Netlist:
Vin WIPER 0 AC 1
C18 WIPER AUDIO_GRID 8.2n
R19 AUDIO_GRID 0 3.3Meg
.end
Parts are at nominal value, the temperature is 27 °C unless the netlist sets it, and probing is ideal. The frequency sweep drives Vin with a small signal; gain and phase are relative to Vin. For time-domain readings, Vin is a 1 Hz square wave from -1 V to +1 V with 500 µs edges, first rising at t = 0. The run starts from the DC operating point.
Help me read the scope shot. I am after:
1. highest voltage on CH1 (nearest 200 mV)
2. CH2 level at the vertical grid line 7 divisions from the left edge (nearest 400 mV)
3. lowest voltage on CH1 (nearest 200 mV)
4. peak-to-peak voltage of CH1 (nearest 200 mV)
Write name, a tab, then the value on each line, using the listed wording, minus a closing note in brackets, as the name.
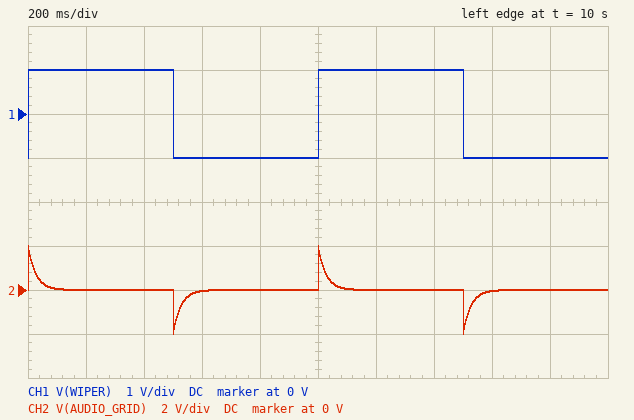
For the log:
highest voltage on CH1	1.0 V
CH2 level at the vertical grid line 7 divisions from the left edge	0 V
lowest voltage on CH1	-1.0 V
peak-to-peak voltage of CH1	2.0 V
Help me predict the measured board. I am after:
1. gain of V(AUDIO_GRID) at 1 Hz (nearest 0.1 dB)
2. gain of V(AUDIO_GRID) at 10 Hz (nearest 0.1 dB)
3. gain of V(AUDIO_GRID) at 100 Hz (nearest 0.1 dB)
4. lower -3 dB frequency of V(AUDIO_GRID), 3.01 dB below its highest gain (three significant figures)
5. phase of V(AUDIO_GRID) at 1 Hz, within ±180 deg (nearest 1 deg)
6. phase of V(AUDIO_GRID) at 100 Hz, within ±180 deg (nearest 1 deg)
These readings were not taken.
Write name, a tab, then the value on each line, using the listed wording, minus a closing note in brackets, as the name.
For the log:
gain of V(AUDIO_GRID) at 1 Hz	-15.5 dB
gain of V(AUDIO_GRID) at 10 Hz	-1.3 dB
gain of V(AUDIO_GRID) at 100 Hz	0 dB
lower -3 dB frequency of V(AUDIO_GRID), 3.01 dB below its highest gain	5.88 Hz
phase of V(AUDIO_GRID) at 1 Hz, within ±180 deg	80 deg
phase of V(AUDIO_GRID) at 100 Hz, within ±180 deg	3 deg
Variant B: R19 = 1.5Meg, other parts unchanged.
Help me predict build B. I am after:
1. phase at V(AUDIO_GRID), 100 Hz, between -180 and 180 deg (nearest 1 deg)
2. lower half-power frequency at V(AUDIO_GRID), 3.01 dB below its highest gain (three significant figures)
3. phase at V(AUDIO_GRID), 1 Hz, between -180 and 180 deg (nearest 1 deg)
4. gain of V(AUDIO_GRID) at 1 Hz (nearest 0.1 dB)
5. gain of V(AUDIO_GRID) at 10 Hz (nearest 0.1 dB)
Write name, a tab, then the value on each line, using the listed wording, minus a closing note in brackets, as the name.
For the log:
phase at V(AUDIO_GRID), 100 Hz, between -180 and 180 deg	7 deg
lower half-power frequency at V(AUDIO_GRID), 3.01 dB below its highest gain	12.9 Hz
phase at V(AUDIO_GRID), 1 Hz, between -180 and 180 deg	86 deg
gain of V(AUDIO_GRID) at 1 Hz	-22.3 dB
gain of V(AUDIO_GRID) at 10 Hz	-4.3 dB
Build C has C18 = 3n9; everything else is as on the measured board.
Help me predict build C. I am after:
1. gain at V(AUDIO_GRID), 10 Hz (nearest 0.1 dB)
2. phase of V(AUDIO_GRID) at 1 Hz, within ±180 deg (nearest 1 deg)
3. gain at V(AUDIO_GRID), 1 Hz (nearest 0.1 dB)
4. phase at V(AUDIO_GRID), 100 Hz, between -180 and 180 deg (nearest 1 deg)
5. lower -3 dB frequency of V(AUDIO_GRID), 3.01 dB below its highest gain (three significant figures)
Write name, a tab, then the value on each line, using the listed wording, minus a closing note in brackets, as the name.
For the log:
gain at V(AUDIO_GRID), 10 Hz	-4.0 dB
phase of V(AUDIO_GRID) at 1 Hz, within ±180 deg	85 deg
gain at V(AUDIO_GRID), 1 Hz	-21.9 dB
phase at V(AUDIO_GRID), 100 Hz, between -180 and 180 deg	7 deg
lower -3 dB frequency of V(AUDIO_GRID), 3.01 dB below its highest gain	12.4 Hz
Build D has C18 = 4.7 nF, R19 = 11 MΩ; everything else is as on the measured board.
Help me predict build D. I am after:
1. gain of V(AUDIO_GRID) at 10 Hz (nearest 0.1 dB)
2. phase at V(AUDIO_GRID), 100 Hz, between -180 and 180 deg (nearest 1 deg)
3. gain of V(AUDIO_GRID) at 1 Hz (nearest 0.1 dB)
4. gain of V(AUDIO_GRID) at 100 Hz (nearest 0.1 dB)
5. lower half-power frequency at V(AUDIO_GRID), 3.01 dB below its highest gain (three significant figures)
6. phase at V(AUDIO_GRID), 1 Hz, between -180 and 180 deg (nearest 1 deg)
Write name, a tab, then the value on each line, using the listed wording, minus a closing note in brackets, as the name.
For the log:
gain of V(AUDIO_GRID) at 10 Hz	-0.4 dB
phase at V(AUDIO_GRID), 100 Hz, between -180 and 180 deg	2 deg
gain of V(AUDIO_GRID) at 1 Hz	-10.2 dB
gain of V(AUDIO_GRID) at 100 Hz	0 dB
lower half-power frequency at V(AUDIO_GRID), 3.01 dB below its highest gain	3.08 Hz
phase at V(AUDIO_GRID), 1 Hz, between -180 and 180 deg	72 deg
